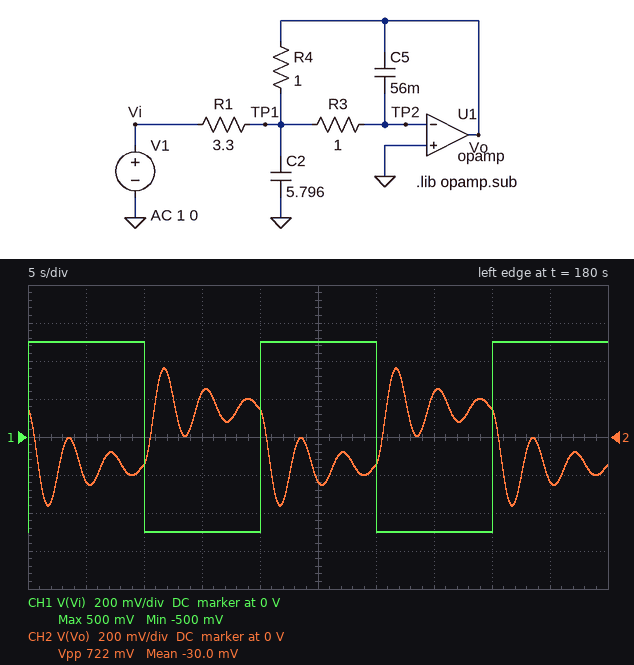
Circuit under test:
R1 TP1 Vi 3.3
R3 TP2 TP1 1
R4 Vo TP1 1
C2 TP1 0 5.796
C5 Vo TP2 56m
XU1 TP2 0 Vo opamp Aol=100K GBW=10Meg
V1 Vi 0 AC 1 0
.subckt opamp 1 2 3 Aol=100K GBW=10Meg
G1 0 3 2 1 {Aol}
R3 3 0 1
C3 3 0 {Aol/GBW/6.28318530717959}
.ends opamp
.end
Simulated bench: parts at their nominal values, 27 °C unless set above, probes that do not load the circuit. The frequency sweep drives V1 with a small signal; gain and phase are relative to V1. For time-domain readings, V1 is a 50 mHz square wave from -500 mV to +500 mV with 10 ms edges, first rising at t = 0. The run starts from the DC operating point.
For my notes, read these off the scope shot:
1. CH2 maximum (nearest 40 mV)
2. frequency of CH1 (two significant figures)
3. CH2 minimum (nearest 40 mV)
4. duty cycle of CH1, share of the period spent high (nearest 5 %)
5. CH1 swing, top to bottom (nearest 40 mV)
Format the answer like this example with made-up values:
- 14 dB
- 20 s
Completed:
- 360 mV
- 50 mHz
- -360 mV
- 50 %
- 1.00 V
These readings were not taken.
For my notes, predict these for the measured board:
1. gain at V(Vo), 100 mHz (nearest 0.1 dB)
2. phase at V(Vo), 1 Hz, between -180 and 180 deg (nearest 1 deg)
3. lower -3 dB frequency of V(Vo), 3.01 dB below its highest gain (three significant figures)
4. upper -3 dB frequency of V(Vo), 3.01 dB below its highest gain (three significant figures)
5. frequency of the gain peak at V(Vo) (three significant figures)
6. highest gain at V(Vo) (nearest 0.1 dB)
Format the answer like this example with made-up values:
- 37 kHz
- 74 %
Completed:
- -9.2 dB
- 4 deg
- 242 mHz
- 306 mHz
- 276 mHz
- 2.6 dB
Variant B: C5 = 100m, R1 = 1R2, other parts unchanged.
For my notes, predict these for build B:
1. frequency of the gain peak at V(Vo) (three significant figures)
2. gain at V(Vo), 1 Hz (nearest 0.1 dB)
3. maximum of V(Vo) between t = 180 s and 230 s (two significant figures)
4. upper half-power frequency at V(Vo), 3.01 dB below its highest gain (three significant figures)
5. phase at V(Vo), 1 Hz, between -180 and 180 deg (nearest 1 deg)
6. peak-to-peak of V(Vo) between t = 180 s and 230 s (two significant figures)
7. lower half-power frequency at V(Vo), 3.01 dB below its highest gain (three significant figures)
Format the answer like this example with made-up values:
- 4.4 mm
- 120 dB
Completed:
- 202 mHz
- -28.4 dB
- 840 mV
- 238 mHz
- 5 deg
- 1.7 V
- 157 mHz
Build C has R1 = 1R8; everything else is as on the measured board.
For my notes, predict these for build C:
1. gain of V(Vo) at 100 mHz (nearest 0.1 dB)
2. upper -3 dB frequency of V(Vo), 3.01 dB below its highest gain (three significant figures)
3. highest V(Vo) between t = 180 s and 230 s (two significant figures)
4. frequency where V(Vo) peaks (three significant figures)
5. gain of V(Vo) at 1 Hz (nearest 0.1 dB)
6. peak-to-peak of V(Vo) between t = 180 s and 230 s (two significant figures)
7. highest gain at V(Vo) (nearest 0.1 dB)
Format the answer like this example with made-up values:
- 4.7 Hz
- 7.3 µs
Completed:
- -4.0 dB
- 308 mHz
- 650 mV
- 275 mHz
- -26.6 dB
- 1.3 V
- 7.0 dB
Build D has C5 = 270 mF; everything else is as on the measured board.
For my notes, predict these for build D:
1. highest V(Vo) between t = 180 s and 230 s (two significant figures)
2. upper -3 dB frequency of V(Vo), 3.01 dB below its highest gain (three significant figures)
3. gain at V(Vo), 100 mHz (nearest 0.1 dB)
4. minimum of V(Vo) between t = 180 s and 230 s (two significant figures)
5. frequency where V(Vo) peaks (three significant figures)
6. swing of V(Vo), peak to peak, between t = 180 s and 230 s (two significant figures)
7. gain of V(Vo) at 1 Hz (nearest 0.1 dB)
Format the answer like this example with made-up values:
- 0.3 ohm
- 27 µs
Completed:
- 280 mV
- 148 mHz
- -5.1 dB
- -280 mV
- 119 mHz
- 560 mV
- -46.1 dB
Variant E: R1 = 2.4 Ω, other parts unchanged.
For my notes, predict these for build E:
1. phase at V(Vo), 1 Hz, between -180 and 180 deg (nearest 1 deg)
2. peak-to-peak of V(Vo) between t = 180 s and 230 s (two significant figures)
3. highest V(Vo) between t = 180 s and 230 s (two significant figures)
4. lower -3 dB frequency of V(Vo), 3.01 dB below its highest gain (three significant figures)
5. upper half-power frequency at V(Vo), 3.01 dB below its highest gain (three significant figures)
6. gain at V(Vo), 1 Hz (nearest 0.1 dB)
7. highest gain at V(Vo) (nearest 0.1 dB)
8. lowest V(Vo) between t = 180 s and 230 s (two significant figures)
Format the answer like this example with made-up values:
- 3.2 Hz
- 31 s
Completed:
- 4 deg
- 980 mV
- 490 mV
- 240 mHz
- 307 mHz
- -29.1 dB
- 4.9 dB
- -490 mV
